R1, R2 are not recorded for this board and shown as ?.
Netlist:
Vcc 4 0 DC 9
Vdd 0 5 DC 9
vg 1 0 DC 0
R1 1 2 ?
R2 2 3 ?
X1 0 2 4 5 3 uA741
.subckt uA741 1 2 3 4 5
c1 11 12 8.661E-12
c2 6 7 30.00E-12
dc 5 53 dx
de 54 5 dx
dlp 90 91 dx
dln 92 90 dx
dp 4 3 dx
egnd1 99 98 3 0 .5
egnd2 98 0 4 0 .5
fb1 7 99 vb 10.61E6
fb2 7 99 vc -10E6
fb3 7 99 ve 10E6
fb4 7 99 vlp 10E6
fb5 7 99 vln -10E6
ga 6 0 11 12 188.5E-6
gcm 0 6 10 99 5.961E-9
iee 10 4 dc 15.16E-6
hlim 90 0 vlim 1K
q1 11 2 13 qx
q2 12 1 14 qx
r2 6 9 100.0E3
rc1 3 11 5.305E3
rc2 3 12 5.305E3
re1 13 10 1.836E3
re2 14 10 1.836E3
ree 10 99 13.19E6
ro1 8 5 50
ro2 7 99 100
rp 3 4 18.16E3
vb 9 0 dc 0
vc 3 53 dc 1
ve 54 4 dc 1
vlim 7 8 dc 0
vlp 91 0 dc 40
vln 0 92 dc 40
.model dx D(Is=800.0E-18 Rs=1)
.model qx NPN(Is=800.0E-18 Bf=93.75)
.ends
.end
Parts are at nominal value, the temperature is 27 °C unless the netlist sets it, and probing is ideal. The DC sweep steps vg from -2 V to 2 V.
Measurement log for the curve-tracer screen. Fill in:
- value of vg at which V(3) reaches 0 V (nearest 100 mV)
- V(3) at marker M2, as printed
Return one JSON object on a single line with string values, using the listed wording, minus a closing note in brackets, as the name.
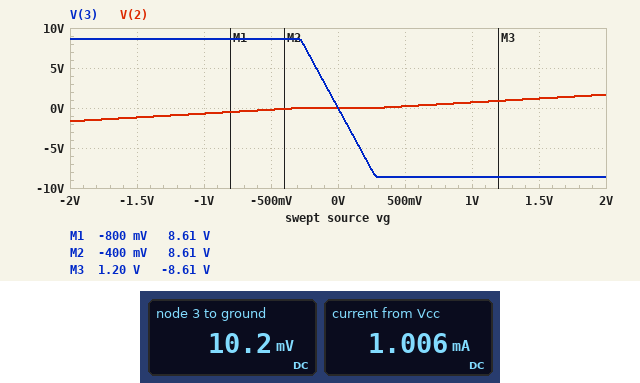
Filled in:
{"value of vg at which V(3) reaches 0 V": "0 V", "V(3) at marker M2, as printed": "8.61 V"}
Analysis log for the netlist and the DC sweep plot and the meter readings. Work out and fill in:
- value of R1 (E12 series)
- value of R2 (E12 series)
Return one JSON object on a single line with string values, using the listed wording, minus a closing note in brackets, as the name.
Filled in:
{"value of R1": "3.9 kΩ", "value of R2": "120 kΩ"}
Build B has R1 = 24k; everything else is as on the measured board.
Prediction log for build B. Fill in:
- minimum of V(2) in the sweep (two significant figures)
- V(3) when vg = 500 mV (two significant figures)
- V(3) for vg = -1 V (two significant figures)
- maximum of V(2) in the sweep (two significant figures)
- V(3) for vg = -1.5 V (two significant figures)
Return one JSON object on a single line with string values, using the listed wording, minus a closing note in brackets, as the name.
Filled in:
{"minimum of V(2) in the sweep": "-230 mV", "V(3) when vg = 500 mV": "-2.5 V", "V(3) for vg = -1 V": "5.0 V", "maximum of V(2) in the sweep": "230 mV", "V(3) for vg = -1.5 V": "7.5 V"}
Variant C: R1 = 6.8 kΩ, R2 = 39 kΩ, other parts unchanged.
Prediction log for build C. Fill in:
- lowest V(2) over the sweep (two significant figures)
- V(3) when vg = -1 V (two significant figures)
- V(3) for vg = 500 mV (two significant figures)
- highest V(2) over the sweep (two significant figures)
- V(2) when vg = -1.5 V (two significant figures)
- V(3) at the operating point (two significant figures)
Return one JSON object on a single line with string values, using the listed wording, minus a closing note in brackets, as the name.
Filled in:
{"lowest V(2) over the sweep": "-420 mV", "V(3) when vg = -1 V": "5.7 V", "V(3) for vg = 500 mV": "-2.9 V", "highest V(2) over the sweep": "420 mV", "V(2) when vg = -1.5 V": "-7.8 mV", "V(3) at the operating point": "3.2 mV"}
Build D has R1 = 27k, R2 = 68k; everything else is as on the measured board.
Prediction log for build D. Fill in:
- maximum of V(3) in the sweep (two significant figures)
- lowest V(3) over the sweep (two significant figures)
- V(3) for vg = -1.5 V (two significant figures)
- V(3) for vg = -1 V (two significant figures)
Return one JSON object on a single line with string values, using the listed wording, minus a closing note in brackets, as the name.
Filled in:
{"maximum of V(3) in the sweep": "5.0 V", "lowest V(3) over the sweep": "-5.0 V", "V(3) for vg = -1.5 V": "3.8 V", "V(3) for vg = -1 V": "2.5 V"}
